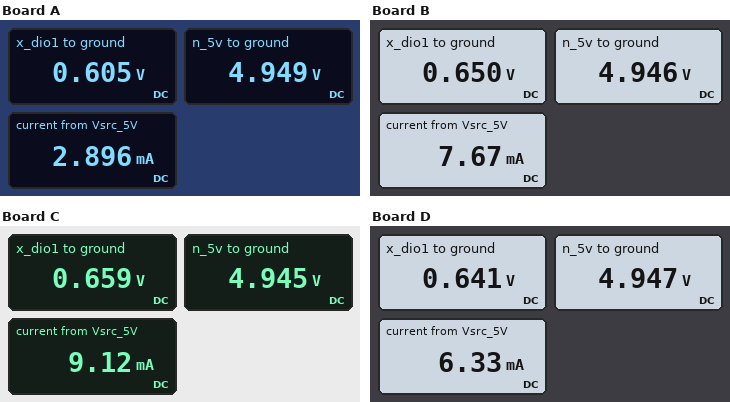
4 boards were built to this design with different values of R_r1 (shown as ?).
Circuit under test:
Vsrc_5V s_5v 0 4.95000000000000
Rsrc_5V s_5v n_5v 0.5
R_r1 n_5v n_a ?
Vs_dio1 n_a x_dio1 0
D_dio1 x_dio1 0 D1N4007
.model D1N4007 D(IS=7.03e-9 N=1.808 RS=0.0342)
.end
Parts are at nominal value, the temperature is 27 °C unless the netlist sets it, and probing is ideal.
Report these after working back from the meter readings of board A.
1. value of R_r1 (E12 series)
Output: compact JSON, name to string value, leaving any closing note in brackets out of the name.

{"value of R_r1": "1.5 kΩ"}
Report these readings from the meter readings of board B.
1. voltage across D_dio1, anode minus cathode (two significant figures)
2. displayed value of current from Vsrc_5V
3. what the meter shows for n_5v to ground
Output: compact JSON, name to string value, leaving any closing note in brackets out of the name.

{"voltage across D_dio1, anode minus cathode": "650 mV", "displayed value of current from Vsrc_5V": "7.67 mA", "what the meter shows for n_5v to ground": "4.946 V"}
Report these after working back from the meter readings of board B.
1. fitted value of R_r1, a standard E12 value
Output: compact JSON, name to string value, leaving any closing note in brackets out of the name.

{"fitted value of R_r1, a standard E12 value": "560 Ω"}
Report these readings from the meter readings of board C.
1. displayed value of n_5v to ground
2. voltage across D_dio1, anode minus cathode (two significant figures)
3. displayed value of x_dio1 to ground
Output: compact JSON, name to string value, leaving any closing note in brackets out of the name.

{"displayed value of n_5v to ground": "4.945 V", "voltage across D_dio1, anode minus cathode": "660 mV", "displayed value of x_dio1 to ground": "0.659 V"}
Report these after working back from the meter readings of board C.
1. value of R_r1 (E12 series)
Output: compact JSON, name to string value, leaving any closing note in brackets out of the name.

{"value of R_r1": "470 Ω"}
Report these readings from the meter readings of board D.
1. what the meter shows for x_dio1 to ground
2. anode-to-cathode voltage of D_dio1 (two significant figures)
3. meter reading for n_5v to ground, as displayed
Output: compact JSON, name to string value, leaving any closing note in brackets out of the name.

{"what the meter shows for x_dio1 to ground": "0.641 V", "anode-to-cathode voltage of D_dio1": "640 mV", "meter reading for n_5v to ground, as displayed": "4.947 V"}
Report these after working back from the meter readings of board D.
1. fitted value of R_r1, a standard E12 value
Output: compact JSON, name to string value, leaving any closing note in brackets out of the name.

{"fitted value of R_r1, a standard E12 value": "680 Ω"}
